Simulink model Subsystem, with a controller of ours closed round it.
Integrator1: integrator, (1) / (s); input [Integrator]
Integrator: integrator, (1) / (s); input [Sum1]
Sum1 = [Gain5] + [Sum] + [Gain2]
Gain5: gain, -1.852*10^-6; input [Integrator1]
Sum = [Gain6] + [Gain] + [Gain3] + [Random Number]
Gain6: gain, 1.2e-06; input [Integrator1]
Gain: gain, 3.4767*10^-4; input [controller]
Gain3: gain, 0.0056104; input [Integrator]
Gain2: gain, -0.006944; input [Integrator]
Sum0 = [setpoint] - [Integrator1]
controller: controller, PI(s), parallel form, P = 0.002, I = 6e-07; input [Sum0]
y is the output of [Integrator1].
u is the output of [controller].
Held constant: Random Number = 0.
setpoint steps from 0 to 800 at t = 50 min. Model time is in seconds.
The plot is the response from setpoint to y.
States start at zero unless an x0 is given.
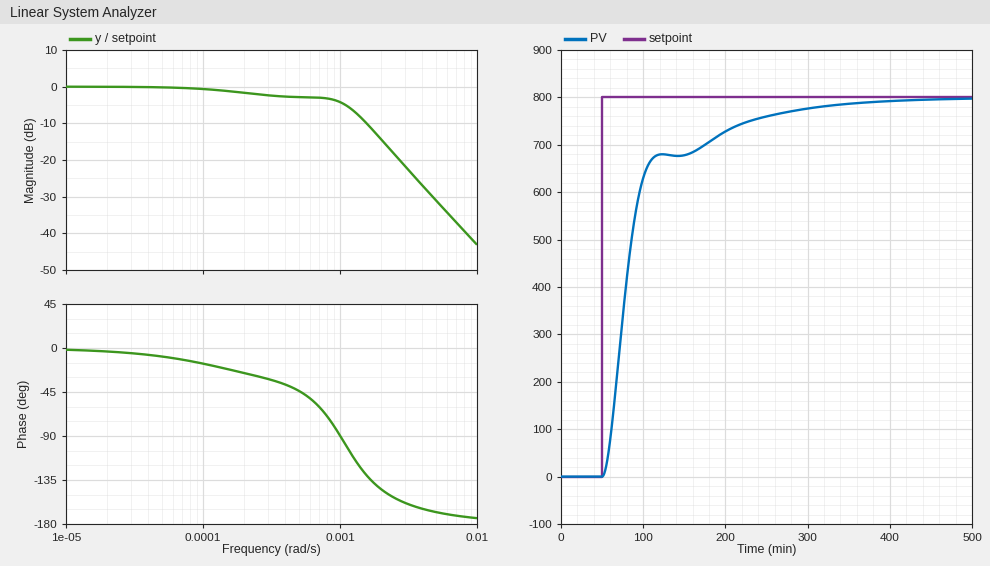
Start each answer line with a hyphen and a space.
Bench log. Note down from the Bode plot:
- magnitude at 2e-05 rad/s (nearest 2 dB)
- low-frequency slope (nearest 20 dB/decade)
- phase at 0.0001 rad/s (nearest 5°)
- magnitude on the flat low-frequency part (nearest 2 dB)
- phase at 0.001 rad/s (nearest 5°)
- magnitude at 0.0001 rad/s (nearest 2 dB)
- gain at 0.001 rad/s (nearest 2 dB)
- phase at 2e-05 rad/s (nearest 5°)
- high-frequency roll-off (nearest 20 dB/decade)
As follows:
- 0 dB
- 0 dB/decade
- -15°
- 0 dB
- -90°
- 0 dB
- -4 dB
- -5°
- -40 dB/decade
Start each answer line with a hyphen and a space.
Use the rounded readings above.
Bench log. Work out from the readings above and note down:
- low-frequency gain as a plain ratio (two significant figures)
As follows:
- 1.0
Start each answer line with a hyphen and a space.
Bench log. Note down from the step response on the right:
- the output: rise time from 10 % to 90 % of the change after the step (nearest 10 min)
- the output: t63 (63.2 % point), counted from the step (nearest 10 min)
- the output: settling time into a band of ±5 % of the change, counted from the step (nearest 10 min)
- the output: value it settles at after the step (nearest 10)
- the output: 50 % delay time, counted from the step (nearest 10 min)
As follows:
- 130 min
- 40 min
- 200 min
- 800
- 30 min
